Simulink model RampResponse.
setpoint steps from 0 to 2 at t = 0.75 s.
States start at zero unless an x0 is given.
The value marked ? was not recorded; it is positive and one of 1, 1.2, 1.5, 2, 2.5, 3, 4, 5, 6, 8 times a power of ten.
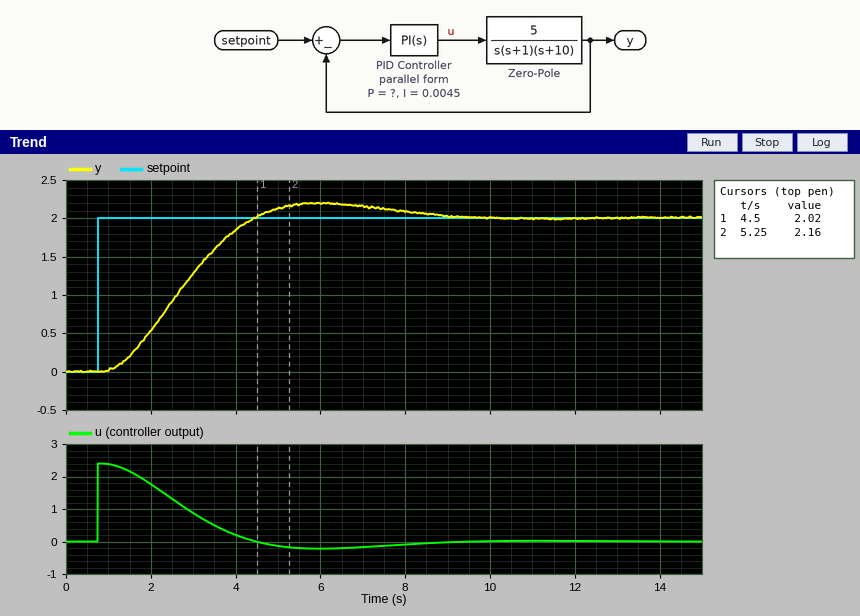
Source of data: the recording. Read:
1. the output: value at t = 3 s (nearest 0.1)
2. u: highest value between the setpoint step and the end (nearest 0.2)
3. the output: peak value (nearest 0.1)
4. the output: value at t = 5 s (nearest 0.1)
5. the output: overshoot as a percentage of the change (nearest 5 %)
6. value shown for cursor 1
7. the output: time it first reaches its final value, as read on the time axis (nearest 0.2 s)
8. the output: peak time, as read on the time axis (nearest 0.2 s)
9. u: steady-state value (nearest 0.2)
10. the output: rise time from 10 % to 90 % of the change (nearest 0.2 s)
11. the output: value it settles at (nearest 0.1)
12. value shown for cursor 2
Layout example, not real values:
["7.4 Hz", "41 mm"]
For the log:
["1.3", "2.4", "2.2", "2.1", "10 %", "2.02", "4.4 s", "6.0 s", "0.0", "2.4 s", "2.0", "2.16"]
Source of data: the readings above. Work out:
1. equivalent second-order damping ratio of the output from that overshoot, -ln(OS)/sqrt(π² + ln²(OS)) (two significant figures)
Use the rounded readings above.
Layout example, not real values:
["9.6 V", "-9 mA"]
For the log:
["0.59"]
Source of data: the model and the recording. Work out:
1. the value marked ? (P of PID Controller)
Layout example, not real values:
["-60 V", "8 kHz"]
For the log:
["1.2"]
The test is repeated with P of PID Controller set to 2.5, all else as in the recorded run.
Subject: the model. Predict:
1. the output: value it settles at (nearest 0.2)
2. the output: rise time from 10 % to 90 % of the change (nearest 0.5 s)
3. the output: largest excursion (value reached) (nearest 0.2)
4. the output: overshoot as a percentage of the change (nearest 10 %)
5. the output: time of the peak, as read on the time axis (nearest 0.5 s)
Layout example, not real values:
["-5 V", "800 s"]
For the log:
["2.0", "1.5 s", "2.6", "30 %", "4.0 s"]
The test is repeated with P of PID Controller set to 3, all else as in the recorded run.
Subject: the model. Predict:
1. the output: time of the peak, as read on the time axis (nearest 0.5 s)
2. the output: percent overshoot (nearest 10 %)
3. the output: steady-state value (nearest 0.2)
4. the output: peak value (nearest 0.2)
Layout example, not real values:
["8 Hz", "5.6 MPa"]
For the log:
["3.5 s", "30 %", "2.0", "2.6"]
